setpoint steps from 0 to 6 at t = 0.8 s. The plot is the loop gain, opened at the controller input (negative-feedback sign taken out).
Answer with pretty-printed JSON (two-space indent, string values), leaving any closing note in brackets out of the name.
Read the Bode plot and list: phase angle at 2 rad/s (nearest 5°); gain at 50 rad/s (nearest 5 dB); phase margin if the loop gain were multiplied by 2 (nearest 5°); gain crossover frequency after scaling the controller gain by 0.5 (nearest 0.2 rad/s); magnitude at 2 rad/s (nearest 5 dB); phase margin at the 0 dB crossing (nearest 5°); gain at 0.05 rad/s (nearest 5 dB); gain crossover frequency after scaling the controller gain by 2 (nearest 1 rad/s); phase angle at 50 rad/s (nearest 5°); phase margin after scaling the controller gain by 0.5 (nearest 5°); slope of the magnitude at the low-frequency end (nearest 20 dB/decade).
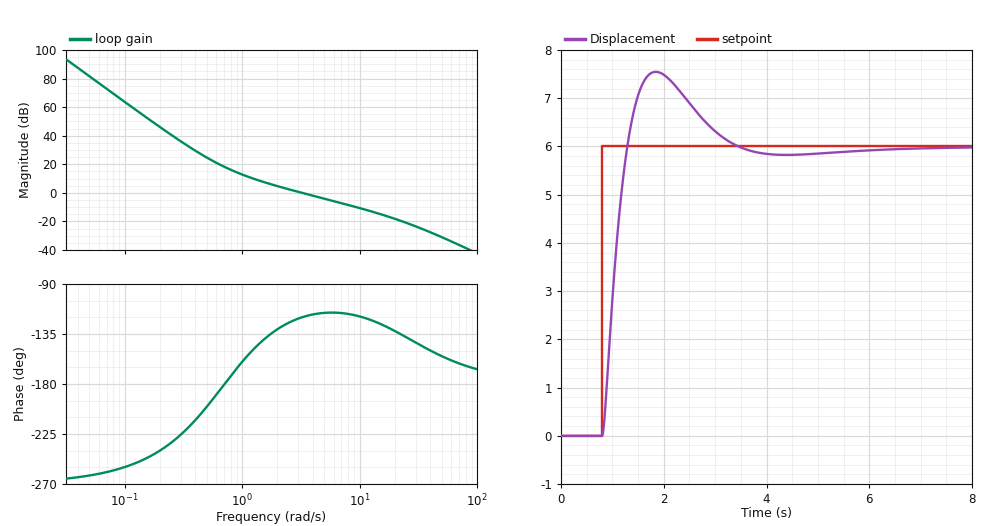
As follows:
{
  "phase angle at 2 rad/s": "-130°",
  "gain at 50 rad/s": "-30 dB",
  "phase margin if the loop gain were multiplied by 2": "65°",
  "gain crossover frequency after scaling the controller gain by 0.5": "1.8 rad/s",
  "magnitude at 2 rad/s": "5 dB",
  "phase margin at the 0 dB crossing": "60°",
  "gain at 0.05 rad/s": "80 dB",
  "gain crossover frequency after scaling the controller gain by 2": "6 rad/s",
  "phase angle at 50 rad/s": "-155°",
  "phase margin after scaling the controller gain by 0.5": "45°",
  "slope of the magnitude at the low-frequency end": "-60 dB/decade"
}
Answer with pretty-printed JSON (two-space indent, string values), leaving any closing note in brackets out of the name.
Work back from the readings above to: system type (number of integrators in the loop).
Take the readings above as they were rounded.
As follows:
{
  "system type": "3"
}
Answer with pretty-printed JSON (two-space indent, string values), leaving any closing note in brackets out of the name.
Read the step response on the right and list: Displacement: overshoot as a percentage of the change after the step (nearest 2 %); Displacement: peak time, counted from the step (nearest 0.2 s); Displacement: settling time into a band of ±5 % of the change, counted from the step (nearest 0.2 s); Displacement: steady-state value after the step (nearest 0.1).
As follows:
{
  "Displacement: overshoot as a percentage of the change after the step": "26 %",
  "Displacement: peak time, counted from the step": "1.0 s",
  "Displacement: settling time into a band of ±5 % of the change, counted from the step": "2.2 s",
  "Displacement: steady-state value after the step": "6.0"
}
